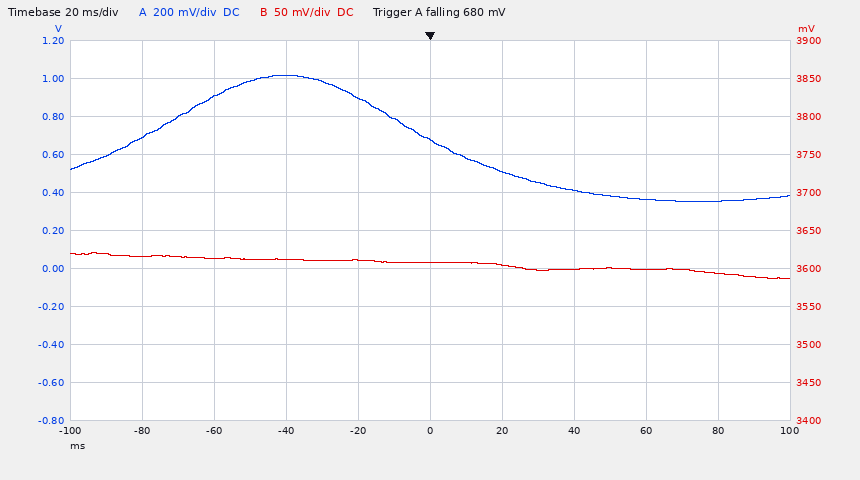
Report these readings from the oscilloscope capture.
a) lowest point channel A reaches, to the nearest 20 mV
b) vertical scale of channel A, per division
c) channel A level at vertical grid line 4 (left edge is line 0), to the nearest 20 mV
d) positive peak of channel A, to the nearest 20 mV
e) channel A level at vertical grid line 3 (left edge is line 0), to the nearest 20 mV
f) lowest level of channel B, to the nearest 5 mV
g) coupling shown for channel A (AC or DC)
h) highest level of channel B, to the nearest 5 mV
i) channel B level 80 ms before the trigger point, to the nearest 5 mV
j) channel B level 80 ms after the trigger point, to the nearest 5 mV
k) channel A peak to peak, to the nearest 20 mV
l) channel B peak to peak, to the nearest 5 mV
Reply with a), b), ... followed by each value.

a) 360 mV
b) 200 mV
c) 900 mV
d) 1.02 V
e) 1.02 V
f) 3.585 V
g) DC
h) 3.620 V
i) 3.615 V
j) 3.595 V
k) 660 mV
l) 35 mV
